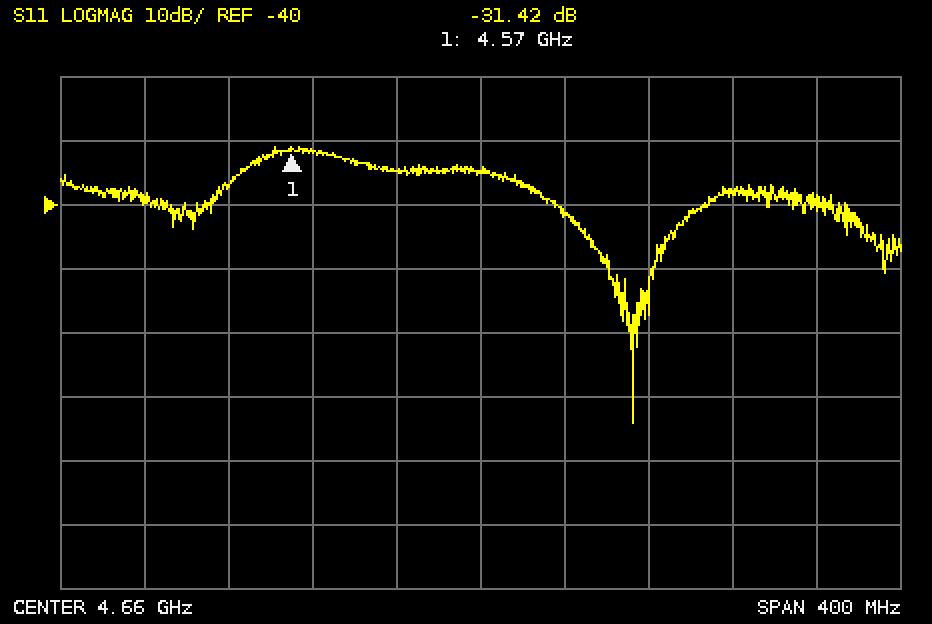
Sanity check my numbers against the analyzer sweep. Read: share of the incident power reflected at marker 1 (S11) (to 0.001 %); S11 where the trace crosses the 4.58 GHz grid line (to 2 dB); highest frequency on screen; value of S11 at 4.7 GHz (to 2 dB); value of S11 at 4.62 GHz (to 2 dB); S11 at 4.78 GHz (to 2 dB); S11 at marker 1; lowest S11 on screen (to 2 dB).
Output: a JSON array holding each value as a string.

["0.072 %", "-32 dB", "4.86 GHz", "-42 dB", "-34 dB", "-38 dB", "-31.42 dB", "-74 dB"]
